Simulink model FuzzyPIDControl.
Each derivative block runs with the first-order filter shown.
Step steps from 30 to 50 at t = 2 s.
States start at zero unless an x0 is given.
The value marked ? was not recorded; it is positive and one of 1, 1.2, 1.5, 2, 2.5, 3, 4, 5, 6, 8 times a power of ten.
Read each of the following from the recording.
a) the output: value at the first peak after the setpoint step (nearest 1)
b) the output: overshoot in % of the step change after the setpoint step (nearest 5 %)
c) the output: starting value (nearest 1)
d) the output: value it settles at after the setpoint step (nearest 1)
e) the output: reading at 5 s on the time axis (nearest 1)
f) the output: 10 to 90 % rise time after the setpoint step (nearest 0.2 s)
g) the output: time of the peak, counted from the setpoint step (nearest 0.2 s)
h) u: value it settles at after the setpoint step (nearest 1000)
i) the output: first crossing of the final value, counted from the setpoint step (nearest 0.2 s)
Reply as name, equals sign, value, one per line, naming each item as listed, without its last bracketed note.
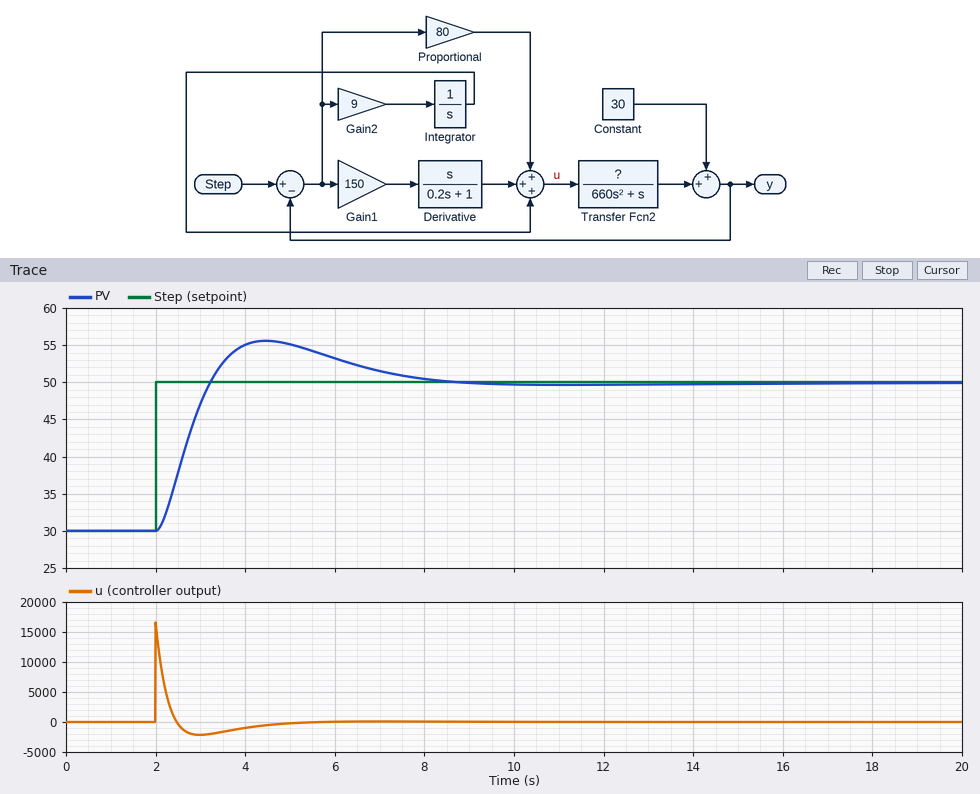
the output: value at the first peak after the setpoint step = 56
the output: overshoot in % of the step change after the setpoint step = 30 %
the output: starting value = 30
the output: value it settles at after the setpoint step = 50
the output: reading at 5 s on the time axis = 55
the output: 10 to 90 % rise time after the setpoint step = 0.8 s
the output: time of the peak, counted from the setpoint step = 2.4 s
u: value it settles at after the setpoint step = 0
the output: first crossing of the final value, counted from the setpoint step = 1.2 s
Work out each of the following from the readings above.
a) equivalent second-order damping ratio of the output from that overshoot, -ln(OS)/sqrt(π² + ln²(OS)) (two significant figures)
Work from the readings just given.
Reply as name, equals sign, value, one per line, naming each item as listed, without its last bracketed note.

equivalent second-order damping ratio of the output from that overshoot, -ln(OS)/sqrt(π² + ln²(OS)) = 0.36
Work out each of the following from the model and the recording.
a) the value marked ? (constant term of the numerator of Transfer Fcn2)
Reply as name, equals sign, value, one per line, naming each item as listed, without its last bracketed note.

the value marked ? = 5
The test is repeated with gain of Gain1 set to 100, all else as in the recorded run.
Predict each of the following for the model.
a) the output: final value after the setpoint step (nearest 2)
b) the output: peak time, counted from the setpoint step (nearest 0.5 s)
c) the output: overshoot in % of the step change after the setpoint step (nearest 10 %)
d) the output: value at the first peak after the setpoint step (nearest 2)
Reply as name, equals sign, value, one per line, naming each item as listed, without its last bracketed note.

the output: final value after the setpoint step = 50
the output: peak time, counted from the setpoint step = 3.0 s
the output: overshoot in % of the step change after the setpoint step = 40 %
the output: value at the first peak after the setpoint step = 58
